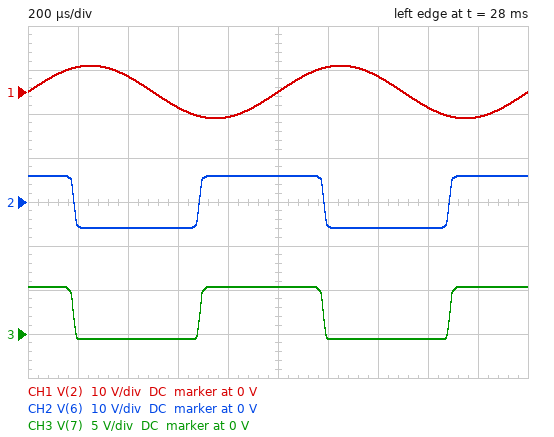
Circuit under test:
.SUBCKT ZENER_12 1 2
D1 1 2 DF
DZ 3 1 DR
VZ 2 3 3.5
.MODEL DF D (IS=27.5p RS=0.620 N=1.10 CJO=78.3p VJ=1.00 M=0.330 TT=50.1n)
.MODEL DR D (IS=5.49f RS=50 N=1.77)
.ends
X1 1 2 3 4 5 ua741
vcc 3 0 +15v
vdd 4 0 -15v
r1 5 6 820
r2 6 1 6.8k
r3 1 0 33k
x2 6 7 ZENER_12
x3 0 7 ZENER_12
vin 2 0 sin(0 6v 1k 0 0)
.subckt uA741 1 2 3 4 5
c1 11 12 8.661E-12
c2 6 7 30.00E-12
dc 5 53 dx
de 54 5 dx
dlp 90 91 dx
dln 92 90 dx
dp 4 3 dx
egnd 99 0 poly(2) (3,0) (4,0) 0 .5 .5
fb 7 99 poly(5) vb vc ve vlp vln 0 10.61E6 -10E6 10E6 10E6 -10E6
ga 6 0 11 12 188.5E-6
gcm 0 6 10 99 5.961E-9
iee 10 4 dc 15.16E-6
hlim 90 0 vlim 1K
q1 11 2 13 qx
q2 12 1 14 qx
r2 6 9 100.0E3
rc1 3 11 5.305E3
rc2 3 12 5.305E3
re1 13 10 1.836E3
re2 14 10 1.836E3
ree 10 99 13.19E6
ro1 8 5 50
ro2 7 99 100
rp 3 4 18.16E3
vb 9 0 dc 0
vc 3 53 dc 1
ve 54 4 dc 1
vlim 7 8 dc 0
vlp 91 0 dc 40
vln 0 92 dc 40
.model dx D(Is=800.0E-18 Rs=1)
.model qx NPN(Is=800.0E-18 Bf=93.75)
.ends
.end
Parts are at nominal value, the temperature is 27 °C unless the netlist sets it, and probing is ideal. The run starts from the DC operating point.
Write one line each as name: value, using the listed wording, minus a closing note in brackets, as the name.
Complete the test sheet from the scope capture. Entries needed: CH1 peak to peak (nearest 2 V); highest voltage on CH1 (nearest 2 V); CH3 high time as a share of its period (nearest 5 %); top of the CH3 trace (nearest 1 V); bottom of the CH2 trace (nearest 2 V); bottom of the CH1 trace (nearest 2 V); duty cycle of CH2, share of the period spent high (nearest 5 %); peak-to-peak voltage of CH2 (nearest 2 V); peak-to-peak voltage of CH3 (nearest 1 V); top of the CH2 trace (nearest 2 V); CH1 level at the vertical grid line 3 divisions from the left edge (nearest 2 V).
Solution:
CH1 peak to peak: 12 V
highest voltage on CH1: 6 V
CH3 high time as a share of its period: 50 %
top of the CH3 trace: 5 V
bottom of the CH2 trace: -6 V
bottom of the CH1 trace: -6 V
duty cycle of CH2, share of the period spent high: 50 %
peak-to-peak voltage of CH2: 12 V
peak-to-peak voltage of CH3: 6 V
top of the CH2 trace: 6 V
CH1 level at the vertical grid line 3 divisions from the left edge: -4 V
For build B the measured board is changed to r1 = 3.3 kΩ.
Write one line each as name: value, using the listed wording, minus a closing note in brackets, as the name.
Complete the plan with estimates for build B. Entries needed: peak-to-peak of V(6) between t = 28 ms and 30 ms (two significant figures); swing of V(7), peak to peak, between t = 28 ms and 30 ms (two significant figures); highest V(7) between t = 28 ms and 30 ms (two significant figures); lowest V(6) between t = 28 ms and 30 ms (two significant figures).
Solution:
peak-to-peak of V(6) between t = 28 ms and 30 ms: 11 V
swing of V(7), peak to peak, between t = 28 ms and 30 ms: 5.4 V
highest V(7) between t = 28 ms and 30 ms: 4.9 V
lowest V(6) between t = 28 ms and 30 ms: -5.4 V
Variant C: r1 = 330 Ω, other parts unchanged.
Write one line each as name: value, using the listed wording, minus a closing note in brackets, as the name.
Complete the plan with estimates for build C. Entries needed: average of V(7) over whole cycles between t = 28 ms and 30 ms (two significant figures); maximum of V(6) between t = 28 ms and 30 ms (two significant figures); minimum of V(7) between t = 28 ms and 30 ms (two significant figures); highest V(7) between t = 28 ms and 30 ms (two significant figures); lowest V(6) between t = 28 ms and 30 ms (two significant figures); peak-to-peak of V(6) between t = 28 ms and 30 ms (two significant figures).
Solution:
average of V(7) over whole cycles between t = 28 ms and 30 ms: 2.6 V
maximum of V(6) between t = 28 ms and 30 ms: 6.6 V
minimum of V(7) between t = 28 ms and 30 ms: -600 mV
highest V(7) between t = 28 ms and 30 ms: 6.0 V
lowest V(6) between t = 28 ms and 30 ms: -6.6 V
peak-to-peak of V(6) between t = 28 ms and 30 ms: 13 V
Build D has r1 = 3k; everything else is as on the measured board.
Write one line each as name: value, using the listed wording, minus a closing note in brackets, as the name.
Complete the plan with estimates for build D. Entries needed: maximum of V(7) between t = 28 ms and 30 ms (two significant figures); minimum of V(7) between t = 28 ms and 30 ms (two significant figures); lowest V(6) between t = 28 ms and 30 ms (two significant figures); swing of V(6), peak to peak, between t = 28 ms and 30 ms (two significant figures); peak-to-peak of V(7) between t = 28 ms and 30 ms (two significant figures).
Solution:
maximum of V(7) between t = 28 ms and 30 ms: 4.9 V
minimum of V(7) between t = 28 ms and 30 ms: -530 mV
lowest V(6) between t = 28 ms and 30 ms: -5.4 V
swing of V(6), peak to peak, between t = 28 ms and 30 ms: 11 V
peak-to-peak of V(7) between t = 28 ms and 30 ms: 5.4 V
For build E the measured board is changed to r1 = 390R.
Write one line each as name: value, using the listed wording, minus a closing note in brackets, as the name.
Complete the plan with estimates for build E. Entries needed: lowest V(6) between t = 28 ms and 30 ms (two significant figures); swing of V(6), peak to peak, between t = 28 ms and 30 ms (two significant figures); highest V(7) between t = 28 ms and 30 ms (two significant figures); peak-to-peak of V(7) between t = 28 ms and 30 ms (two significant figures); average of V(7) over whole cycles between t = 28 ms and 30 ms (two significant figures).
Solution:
lowest V(6) between t = 28 ms and 30 ms: -6.5 V
swing of V(6), peak to peak, between t = 28 ms and 30 ms: 13 V
highest V(7) between t = 28 ms and 30 ms: 5.9 V
peak-to-peak of V(7) between t = 28 ms and 30 ms: 6.5 V
average of V(7) over whole cycles between t = 28 ms and 30 ms: 2.6 V
